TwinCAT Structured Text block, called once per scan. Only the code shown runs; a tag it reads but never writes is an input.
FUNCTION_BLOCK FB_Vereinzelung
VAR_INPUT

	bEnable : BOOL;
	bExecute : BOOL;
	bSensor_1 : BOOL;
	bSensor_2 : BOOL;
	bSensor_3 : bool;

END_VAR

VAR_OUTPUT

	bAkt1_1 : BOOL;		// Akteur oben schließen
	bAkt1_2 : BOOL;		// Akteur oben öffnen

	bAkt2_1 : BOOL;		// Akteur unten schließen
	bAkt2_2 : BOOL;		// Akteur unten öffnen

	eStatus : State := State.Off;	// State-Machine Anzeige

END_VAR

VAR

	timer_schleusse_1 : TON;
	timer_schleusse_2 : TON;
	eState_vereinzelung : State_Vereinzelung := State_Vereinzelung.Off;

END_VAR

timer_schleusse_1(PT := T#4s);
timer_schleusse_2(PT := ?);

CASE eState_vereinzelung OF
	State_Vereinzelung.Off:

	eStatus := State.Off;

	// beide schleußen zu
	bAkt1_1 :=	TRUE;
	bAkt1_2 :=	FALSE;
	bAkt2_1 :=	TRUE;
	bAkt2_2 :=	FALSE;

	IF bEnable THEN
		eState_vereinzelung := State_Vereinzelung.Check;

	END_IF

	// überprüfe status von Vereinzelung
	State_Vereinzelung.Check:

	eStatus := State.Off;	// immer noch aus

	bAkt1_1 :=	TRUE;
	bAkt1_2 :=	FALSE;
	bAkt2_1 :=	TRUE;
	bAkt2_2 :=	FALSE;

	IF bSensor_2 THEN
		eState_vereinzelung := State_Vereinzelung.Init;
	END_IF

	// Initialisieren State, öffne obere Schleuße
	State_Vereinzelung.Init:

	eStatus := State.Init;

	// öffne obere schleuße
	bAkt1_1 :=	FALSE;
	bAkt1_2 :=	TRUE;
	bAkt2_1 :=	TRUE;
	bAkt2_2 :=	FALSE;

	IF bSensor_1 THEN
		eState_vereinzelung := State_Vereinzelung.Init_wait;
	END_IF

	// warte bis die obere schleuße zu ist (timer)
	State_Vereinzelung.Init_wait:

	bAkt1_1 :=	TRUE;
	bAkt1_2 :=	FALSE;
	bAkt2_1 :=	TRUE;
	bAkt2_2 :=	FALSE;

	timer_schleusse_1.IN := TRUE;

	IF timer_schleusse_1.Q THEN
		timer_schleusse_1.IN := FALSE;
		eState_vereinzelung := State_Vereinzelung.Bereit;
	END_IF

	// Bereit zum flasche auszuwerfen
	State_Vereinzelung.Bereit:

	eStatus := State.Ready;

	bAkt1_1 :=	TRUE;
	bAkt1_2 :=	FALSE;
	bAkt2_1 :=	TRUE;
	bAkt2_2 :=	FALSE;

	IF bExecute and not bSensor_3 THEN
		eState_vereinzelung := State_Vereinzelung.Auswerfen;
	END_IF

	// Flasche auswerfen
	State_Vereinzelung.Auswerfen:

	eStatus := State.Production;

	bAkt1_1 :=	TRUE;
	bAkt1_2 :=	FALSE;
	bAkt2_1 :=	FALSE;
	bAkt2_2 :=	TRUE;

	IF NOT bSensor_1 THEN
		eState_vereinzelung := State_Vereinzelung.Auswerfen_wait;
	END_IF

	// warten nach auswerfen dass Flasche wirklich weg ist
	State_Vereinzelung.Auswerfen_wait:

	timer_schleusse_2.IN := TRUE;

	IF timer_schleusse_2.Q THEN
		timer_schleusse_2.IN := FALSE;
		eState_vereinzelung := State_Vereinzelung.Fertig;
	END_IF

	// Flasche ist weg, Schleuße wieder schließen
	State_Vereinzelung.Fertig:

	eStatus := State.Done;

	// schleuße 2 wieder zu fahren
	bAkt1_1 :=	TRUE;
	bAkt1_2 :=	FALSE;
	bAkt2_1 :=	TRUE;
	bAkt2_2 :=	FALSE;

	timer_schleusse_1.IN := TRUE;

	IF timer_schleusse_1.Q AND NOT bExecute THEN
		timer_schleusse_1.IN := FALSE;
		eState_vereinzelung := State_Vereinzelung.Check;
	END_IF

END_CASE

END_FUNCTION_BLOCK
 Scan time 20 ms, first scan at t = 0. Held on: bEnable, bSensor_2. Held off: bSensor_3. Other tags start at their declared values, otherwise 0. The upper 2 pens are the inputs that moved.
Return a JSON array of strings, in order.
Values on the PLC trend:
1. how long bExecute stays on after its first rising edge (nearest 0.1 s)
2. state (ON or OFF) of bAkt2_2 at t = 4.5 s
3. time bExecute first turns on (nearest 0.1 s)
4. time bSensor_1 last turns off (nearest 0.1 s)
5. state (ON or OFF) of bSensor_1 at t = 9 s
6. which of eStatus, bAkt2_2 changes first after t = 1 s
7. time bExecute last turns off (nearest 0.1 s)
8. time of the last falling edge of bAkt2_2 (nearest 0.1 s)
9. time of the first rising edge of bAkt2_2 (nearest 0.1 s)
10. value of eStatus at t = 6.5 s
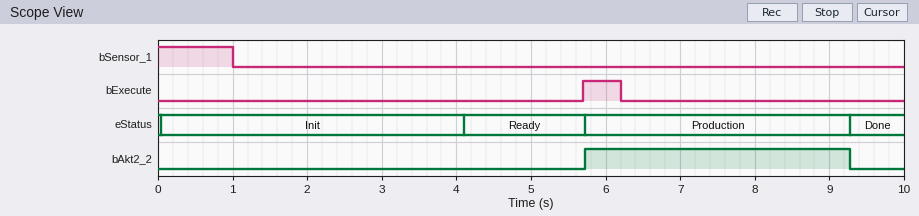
["0.5 s", "OFF", "5.7 s", "1.0 s", "OFF", "eStatus", "6.2 s", "9.3 s", "5.7 s", "Production"]
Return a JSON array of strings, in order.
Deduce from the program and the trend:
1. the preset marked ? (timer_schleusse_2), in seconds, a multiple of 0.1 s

["3.5 s"]
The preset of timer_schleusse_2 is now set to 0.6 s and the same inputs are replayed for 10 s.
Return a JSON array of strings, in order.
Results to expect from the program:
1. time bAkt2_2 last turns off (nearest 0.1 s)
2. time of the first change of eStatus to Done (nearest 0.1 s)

["6.4 s", "6.4 s"]
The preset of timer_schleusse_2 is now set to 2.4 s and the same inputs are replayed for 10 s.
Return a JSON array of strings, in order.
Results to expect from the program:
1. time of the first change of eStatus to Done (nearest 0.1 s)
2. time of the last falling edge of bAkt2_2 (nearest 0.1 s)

["8.2 s", "8.2 s"]
